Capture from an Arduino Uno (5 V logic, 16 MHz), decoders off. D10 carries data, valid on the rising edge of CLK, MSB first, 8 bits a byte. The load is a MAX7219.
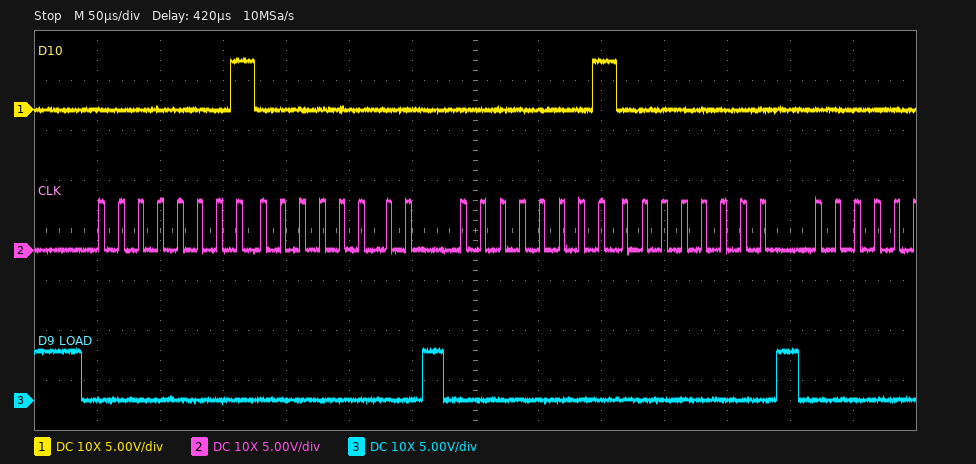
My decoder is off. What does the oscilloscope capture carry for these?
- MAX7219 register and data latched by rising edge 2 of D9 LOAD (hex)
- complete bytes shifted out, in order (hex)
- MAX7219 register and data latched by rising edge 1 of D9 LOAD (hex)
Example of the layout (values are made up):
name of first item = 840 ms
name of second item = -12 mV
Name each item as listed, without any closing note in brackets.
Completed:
MAX7219 register and data latched by rising edge 2 of D9 LOAD = register 0x1, data 0x00
complete bytes shifted out, in order = 01 00 01 00
MAX7219 register and data latched by rising edge 1 of D9 LOAD = register 0x1, data 0x00
